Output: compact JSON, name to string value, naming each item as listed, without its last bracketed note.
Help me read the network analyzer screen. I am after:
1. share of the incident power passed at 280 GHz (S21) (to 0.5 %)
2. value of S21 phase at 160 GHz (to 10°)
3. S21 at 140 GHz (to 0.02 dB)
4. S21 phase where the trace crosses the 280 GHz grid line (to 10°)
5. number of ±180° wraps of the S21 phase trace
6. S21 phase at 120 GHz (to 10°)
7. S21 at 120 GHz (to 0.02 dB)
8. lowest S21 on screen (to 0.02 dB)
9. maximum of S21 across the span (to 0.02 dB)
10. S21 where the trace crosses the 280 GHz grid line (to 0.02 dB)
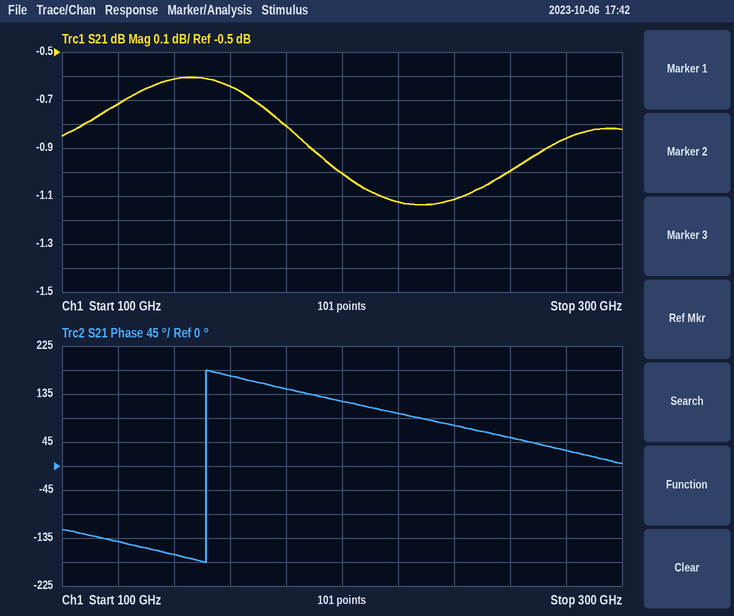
{"share of the incident power passed at 280 GHz (S21)": "82.0 %", "value of S21 phase at 160 GHz": "170°", "S21 at 140 GHz": "-0.62 dB", "S21 phase where the trace crosses the 280 GHz grid line": "30°", "number of ±180° wraps of the S21 phase trace": "1", "S21 phase at 120 GHz": "-140°", "S21 at 120 GHz": "-0.72 dB", "lowest S21 on screen": "-1.14 dB", "maximum of S21 across the span": "-0.60 dB", "S21 where the trace crosses the 280 GHz grid line": "-0.86 dB"}
